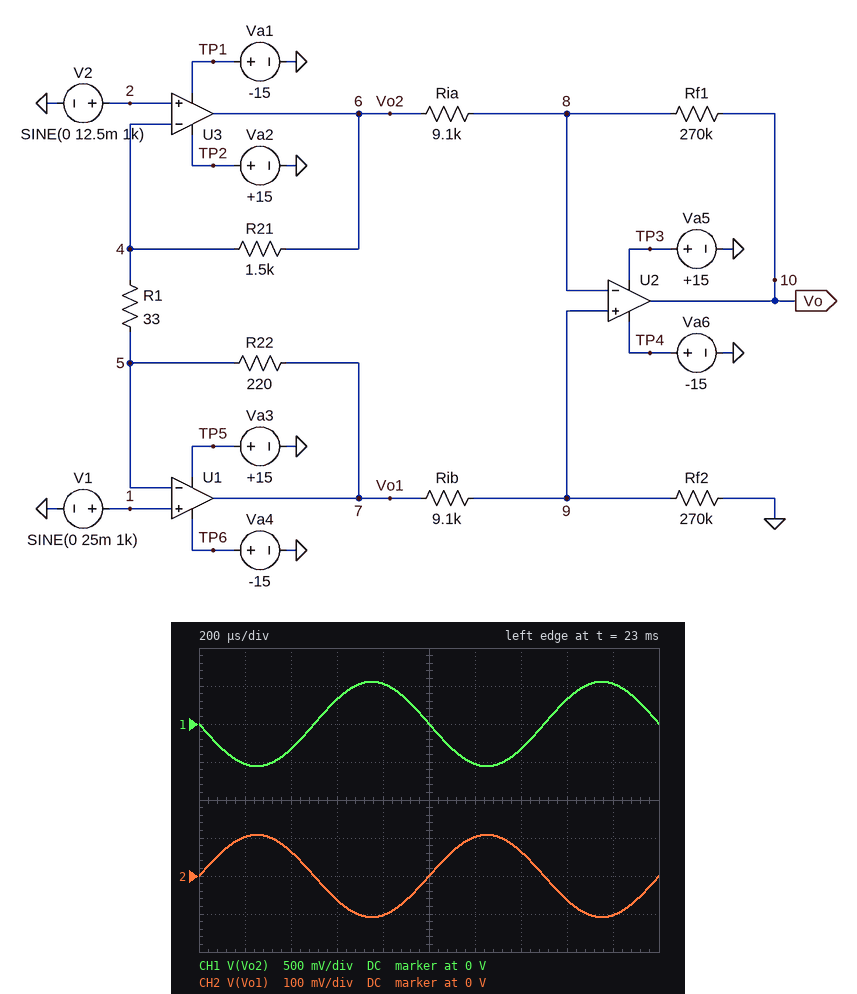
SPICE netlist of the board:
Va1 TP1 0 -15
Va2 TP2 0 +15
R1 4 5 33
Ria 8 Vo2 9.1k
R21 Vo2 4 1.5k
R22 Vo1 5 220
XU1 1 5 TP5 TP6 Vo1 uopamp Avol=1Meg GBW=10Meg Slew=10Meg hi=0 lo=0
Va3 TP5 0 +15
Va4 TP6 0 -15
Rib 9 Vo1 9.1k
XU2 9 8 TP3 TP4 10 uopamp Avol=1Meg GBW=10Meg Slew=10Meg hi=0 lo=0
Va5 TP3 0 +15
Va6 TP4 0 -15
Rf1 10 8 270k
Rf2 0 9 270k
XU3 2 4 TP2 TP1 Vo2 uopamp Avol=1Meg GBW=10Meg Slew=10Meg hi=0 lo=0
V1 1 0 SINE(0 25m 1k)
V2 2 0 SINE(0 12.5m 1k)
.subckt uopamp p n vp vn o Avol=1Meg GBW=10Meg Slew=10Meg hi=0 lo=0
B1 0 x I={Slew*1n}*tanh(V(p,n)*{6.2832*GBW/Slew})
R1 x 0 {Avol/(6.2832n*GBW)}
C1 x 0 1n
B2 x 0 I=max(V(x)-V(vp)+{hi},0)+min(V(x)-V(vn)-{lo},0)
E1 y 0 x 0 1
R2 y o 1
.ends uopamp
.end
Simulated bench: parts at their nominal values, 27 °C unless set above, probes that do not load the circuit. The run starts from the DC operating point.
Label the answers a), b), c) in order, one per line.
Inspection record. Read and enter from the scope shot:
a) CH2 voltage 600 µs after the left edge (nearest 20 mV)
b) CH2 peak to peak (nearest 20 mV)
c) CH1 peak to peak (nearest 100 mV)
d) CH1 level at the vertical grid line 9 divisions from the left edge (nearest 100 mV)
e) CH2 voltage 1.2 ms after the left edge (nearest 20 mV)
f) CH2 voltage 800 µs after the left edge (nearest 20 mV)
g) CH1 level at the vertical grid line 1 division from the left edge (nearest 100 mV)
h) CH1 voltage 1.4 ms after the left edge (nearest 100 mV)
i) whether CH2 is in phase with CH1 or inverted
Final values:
a) -60 mV
b) 220 mV
c) 1.1 V
d) 500 mV
e) 100 mV
f) -100 mV
g) -500 mV
h) -300 mV
i) inverted
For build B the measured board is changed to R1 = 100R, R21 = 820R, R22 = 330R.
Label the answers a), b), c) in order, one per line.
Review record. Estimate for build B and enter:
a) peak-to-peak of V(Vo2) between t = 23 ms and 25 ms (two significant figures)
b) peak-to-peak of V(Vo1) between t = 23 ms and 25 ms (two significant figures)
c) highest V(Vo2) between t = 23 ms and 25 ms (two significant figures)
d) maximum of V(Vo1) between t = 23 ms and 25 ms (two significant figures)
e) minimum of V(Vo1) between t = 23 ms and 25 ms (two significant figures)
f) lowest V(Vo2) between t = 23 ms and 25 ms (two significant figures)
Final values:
a) 180 mV
b) 130 mV
c) 90 mV
d) 66 mV
e) -66 mV
f) -90 mV
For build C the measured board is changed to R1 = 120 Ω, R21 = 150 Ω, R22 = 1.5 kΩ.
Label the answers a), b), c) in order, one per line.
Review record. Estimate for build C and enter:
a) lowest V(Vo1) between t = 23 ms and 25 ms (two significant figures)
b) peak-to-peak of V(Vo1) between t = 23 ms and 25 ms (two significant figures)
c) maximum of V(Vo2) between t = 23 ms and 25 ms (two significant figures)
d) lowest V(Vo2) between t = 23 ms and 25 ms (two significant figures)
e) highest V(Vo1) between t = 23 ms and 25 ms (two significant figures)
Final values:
a) -180 mV
b) 360 mV
c) 3.1 mV
d) -3.1 mV
e) 180 mV
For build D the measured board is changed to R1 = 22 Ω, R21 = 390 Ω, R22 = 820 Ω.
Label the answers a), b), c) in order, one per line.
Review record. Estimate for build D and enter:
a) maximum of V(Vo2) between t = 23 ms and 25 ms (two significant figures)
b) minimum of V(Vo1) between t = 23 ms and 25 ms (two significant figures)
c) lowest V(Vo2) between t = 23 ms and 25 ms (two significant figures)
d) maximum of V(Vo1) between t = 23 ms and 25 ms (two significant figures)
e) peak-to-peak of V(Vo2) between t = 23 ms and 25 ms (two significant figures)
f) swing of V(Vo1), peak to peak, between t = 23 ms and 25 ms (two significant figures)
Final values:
a) 210 mV
b) -490 mV
c) -210 mV
d) 490 mV
e) 420 mV
f) 980 mV
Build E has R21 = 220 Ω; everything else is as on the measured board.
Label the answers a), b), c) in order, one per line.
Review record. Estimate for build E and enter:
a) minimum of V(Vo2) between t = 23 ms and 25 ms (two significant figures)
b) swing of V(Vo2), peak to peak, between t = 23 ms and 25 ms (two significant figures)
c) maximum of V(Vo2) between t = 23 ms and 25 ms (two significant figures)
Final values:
a) -71 mV
b) 140 mV
c) 71 mV
